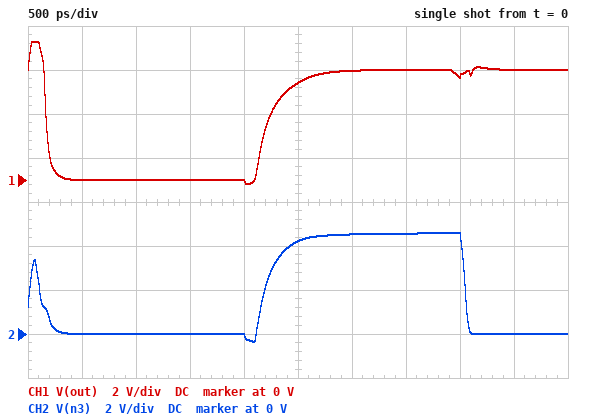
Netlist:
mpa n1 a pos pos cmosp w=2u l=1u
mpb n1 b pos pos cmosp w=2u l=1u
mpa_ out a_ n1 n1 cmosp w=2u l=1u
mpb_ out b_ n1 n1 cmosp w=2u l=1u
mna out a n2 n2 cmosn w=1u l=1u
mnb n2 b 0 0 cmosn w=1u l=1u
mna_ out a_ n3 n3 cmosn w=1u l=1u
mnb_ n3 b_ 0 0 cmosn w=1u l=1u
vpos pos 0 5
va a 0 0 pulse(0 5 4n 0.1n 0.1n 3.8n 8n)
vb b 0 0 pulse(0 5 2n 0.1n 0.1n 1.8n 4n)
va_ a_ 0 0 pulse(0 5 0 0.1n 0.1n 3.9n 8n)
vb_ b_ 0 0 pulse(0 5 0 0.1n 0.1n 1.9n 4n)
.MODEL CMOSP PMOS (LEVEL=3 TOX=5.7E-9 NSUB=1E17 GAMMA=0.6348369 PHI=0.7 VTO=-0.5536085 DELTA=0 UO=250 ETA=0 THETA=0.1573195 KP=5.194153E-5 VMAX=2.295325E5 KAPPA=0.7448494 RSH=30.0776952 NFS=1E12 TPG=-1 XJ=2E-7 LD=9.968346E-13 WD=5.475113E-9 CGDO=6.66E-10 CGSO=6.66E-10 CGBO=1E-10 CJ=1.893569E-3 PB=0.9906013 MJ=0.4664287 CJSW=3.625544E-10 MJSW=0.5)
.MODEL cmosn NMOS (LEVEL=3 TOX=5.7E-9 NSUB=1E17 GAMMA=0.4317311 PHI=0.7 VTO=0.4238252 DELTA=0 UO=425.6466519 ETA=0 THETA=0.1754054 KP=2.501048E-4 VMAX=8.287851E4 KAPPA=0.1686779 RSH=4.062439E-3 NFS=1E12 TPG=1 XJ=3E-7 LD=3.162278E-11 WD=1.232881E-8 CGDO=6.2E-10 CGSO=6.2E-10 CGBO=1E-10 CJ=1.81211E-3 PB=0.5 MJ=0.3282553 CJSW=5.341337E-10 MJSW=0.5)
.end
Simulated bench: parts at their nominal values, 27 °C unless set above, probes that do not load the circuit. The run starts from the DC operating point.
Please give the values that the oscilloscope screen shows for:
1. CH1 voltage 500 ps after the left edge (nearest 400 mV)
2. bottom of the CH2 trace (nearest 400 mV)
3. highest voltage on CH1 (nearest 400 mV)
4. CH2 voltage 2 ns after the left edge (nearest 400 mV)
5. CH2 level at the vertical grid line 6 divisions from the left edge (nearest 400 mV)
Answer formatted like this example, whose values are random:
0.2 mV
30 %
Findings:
0 V
-400 mV
6.4 V
0 V
4.4 V
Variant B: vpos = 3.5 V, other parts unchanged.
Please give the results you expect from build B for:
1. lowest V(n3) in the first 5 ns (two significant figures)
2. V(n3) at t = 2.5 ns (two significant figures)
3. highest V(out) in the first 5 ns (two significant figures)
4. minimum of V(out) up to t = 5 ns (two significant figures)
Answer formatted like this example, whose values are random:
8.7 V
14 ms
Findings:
-590 mV
2.6 V
4.8 V
-380 mV
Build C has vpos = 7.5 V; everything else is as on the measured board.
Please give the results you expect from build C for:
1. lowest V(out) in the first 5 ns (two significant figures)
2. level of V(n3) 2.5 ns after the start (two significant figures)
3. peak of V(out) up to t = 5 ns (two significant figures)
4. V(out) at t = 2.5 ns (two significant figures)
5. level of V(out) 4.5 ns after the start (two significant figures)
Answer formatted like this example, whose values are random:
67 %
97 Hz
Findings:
600 mV
4.5 V
8.8 V
7.4 V
7.5 V
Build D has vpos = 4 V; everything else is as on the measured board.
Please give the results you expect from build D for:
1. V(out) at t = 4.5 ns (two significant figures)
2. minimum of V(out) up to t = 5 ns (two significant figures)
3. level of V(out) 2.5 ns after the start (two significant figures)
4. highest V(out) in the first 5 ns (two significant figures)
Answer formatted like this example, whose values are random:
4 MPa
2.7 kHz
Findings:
4.0 V
-300 mV
3.2 V
5.3 V
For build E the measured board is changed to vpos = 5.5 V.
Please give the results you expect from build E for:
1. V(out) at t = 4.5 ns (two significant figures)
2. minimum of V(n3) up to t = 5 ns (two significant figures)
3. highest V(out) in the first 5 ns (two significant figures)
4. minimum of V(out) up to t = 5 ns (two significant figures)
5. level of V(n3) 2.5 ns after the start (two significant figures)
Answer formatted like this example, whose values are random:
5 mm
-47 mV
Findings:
5.5 V
-270 mV
6.8 V
-160 mV
4.4 V
